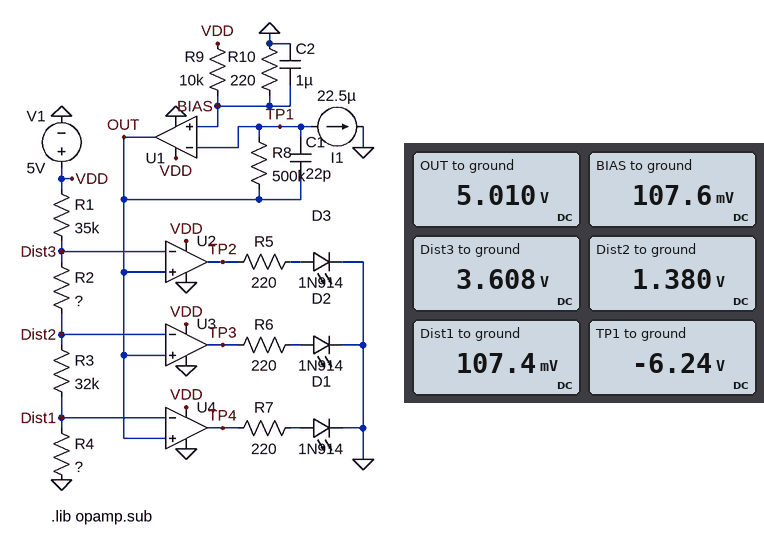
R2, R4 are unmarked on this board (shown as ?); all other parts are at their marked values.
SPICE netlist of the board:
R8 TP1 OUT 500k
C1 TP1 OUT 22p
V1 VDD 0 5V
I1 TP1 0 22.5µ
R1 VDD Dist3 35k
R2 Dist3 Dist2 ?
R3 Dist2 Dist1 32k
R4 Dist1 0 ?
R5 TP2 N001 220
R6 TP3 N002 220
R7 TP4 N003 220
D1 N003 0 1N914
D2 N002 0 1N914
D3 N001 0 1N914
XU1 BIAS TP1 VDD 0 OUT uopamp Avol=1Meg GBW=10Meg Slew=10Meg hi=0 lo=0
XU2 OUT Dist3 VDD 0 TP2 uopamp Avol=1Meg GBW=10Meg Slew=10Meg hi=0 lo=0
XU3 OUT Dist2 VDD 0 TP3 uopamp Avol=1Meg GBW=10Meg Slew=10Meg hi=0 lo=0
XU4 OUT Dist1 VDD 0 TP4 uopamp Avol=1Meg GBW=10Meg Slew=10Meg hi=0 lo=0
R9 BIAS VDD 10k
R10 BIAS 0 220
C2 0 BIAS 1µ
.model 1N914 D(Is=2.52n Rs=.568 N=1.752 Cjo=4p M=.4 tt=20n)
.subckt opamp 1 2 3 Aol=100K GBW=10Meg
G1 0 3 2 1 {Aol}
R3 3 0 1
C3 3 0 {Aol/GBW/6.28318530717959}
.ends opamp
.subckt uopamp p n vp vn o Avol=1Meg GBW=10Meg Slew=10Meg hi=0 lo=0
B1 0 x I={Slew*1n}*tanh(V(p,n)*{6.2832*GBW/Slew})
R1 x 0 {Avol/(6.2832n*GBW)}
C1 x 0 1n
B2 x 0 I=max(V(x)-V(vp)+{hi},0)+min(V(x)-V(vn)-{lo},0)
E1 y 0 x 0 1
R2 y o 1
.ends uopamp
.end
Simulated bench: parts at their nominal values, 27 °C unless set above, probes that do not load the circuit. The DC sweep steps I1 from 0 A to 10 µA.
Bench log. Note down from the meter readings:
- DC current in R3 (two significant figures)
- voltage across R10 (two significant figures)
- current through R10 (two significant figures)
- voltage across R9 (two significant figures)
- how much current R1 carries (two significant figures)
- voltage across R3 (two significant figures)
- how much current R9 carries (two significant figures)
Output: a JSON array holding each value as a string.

["40 µA", "110 mV", "490 µA", "4.9 V", "40 µA", "1.3 V", "490 µA"]
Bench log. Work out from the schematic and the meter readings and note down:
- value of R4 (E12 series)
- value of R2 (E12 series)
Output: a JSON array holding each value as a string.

["2.7 kΩ", "56 kΩ"]
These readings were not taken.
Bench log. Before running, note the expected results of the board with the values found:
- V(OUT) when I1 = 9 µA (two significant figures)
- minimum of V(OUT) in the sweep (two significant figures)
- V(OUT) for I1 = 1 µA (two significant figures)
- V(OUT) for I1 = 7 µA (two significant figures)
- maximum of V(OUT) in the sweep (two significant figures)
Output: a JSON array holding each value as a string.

["4.6 V", "110 mV", "610 mV", "3.6 V", "5.0 V"]
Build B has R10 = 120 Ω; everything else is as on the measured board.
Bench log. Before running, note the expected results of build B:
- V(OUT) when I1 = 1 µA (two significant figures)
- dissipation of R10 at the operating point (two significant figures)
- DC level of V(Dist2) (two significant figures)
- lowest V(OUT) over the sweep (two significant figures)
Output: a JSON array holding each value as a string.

["560 mV", "29 µW", "1.4 V", "59 mV"]
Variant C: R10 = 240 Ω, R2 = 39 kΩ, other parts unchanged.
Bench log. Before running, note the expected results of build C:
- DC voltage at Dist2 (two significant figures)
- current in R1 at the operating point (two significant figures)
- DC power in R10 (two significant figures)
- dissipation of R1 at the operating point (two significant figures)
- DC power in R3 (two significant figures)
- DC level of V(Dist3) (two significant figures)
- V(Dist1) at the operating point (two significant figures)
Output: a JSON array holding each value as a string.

["1.6 V", "46 µA", "57 µW", "74 µW", "68 µW", "3.4 V", "120 mV"]
